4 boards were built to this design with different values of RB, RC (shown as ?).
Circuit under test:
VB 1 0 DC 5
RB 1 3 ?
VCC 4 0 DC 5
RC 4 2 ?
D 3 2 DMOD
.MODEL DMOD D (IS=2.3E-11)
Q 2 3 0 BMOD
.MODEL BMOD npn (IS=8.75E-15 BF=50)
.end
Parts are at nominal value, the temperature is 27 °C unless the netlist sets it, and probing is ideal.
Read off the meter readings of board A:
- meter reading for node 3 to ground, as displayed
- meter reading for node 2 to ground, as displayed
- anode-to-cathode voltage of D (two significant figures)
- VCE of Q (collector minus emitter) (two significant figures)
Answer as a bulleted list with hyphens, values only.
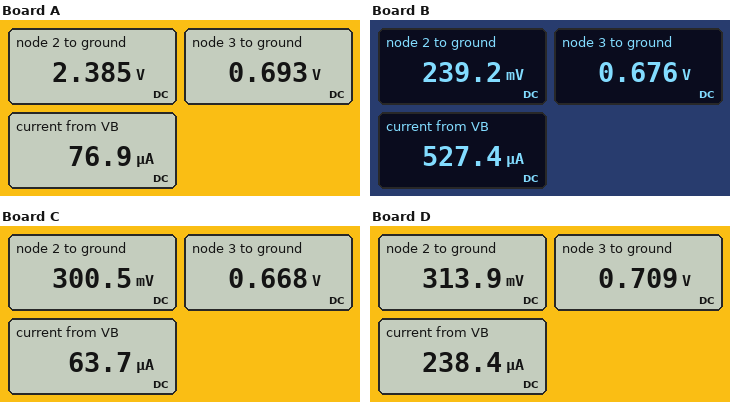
- 0.693 V
- 2.385 V
- -1.7 V
- 2.4 V
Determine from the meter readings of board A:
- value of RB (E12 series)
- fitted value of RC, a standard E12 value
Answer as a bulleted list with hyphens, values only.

- 56 kΩ
- 680 Ω
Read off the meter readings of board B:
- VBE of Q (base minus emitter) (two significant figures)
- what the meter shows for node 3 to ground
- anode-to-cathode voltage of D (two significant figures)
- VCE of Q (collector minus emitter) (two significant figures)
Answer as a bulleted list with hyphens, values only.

- 680 mV
- 0.676 V
- 440 mV
- 240 mV
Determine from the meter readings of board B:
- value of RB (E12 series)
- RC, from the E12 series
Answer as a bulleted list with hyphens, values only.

- 8.2 kΩ
- 3.3 kΩ
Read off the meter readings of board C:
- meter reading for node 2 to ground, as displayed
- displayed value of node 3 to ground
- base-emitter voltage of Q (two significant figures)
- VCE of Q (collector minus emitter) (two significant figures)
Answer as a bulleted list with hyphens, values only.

- 300.5 mV
- 0.668 V
- 670 mV
- 300 mV
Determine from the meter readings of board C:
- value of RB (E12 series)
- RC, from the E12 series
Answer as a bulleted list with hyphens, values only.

- 68 kΩ
- 3.3 kΩ
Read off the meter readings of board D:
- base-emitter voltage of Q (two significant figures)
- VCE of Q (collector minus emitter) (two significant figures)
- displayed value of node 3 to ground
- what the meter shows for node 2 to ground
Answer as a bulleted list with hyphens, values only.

- 710 mV
- 310 mV
- 0.709 V
- 313.9 mV
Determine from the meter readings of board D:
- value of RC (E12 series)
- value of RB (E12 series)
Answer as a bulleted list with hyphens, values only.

- 680 Ω
- 18 kΩ
